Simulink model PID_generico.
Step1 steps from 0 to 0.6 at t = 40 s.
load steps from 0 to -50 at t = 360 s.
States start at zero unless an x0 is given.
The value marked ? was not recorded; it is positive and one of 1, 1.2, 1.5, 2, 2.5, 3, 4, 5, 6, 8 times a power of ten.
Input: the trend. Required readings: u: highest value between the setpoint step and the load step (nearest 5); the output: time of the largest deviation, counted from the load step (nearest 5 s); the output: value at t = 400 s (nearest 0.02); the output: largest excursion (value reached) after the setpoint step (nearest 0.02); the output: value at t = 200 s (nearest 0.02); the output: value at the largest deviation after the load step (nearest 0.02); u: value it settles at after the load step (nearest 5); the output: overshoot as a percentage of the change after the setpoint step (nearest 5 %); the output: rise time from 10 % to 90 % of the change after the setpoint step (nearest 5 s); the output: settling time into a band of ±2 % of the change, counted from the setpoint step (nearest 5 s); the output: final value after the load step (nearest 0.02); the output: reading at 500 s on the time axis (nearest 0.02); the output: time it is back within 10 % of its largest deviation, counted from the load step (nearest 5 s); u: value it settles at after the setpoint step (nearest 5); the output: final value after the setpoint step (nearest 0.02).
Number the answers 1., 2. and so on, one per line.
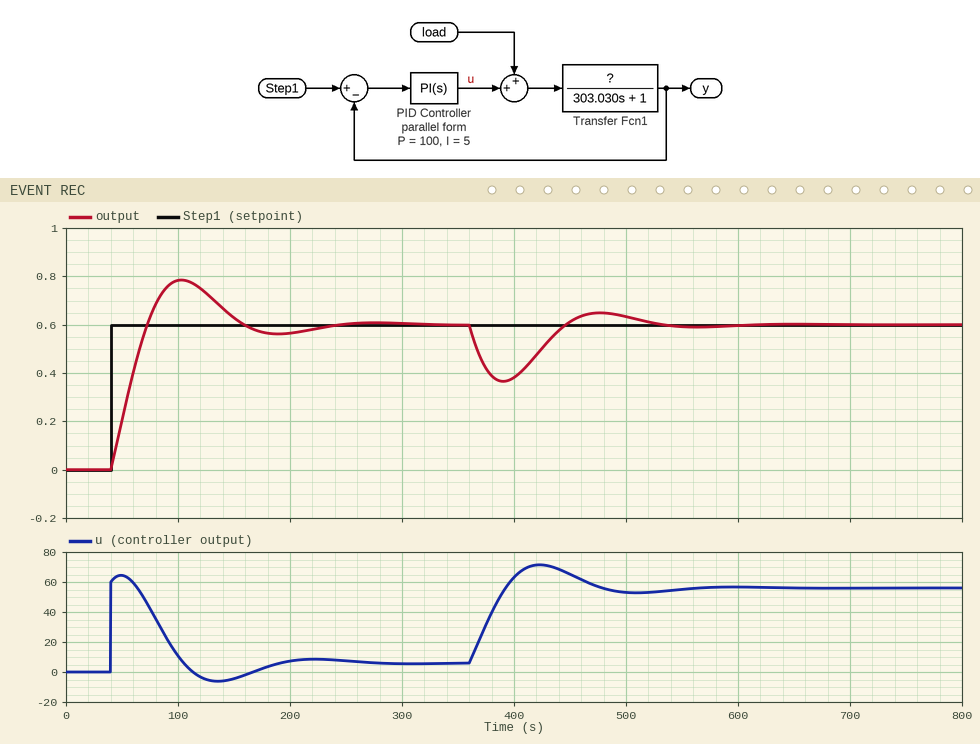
1. 65
2. 30 s
3. 0.38
4. 0.78
5. 0.56
6. 0.36
7. 55
8. 30 %
9. 25 s
10. 190 s
11. 0.60
12. 0.64
13. 150 s
14. 5
15. 0.60
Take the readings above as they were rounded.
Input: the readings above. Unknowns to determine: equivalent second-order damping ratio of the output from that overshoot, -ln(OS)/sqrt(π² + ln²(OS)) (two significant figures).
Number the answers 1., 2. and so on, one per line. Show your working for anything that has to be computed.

1. ln(0.3) = -1.204; 1.204 / sqrt(9.870 + 1.450) = 0.36
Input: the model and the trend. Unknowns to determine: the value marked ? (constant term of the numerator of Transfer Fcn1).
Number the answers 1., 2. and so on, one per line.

1. 0.1
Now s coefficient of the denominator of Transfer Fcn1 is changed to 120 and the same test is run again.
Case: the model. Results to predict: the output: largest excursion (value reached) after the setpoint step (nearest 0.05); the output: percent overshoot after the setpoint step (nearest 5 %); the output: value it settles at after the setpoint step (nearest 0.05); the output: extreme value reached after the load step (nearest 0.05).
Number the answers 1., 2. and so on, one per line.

1. 0.70
2. 15 %
3. 0.60
4. 0.30
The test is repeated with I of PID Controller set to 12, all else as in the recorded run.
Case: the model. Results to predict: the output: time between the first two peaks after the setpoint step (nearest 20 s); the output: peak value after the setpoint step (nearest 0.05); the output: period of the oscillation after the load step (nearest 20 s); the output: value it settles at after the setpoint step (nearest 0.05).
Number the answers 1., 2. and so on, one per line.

1. 100 s
2. 0.85
3. 100 s
4. 0.60
